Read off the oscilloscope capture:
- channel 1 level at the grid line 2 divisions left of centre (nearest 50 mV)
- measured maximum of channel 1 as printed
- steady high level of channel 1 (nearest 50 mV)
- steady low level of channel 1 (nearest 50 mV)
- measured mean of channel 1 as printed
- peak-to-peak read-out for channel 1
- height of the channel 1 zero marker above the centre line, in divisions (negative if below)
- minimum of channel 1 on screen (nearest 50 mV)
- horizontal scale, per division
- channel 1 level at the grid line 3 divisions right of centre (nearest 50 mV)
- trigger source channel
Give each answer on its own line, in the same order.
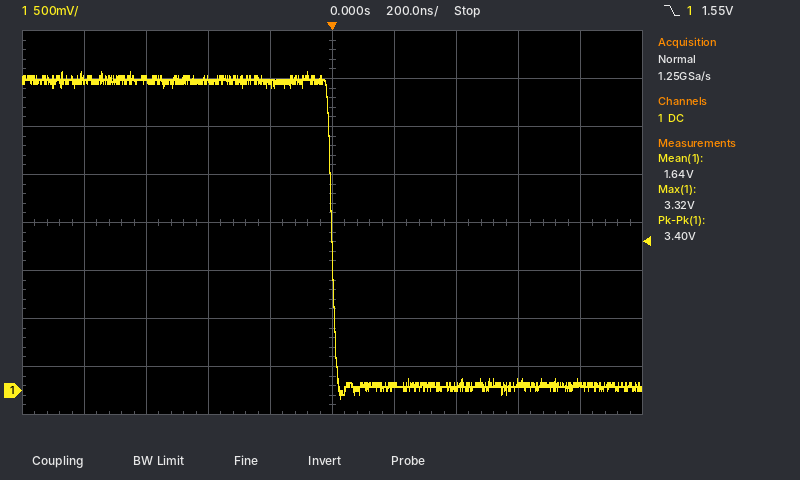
3.25 V
3.32 V
3.25 V
50 mV
1.64 V
3.40 V
-3.5 div
-100 mV
200 ns
100 mV
channel 1
